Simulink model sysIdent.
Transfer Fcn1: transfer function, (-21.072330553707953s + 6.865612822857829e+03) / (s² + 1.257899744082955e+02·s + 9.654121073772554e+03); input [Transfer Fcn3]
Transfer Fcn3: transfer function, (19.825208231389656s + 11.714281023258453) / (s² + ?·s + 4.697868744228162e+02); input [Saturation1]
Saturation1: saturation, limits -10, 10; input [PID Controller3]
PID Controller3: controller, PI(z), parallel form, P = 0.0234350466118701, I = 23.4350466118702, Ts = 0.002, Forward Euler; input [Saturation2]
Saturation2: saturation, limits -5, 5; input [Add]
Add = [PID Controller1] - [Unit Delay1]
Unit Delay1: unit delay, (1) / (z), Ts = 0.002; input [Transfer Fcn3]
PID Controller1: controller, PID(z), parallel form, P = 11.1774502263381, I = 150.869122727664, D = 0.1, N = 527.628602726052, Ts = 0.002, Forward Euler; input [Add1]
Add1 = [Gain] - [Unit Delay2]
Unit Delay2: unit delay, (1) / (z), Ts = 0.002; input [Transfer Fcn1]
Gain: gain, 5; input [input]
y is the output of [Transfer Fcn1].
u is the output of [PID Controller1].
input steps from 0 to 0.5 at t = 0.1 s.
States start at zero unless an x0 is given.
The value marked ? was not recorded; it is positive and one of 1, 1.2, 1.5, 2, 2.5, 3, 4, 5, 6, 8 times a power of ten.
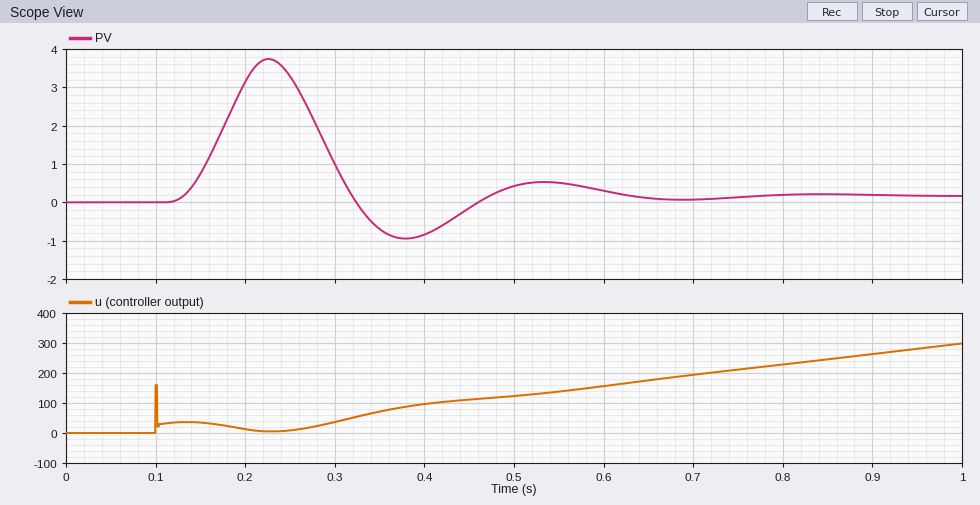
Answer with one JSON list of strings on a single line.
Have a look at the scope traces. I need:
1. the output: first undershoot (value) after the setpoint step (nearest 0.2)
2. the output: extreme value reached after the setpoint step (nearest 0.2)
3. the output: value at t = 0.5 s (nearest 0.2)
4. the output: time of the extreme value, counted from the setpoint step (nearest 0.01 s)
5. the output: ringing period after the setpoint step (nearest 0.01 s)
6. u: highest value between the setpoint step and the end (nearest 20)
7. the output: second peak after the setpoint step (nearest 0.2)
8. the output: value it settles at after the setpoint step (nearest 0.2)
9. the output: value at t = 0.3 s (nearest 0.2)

["-1.0", "3.8", "0.4", "0.13 s", "0.31 s", "300", "0.6", "0.2", "1.0"]
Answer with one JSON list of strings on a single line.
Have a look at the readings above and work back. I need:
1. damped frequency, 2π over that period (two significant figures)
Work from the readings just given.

["20 rad/s"]
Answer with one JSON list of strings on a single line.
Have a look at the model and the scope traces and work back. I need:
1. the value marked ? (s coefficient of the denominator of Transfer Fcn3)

["15"]
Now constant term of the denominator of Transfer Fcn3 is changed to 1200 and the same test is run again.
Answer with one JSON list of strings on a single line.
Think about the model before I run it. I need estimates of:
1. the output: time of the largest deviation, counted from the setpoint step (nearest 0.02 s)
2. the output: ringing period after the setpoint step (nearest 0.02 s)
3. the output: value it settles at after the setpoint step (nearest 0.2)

["0.10 s", "0.18 s", "0.0"]
